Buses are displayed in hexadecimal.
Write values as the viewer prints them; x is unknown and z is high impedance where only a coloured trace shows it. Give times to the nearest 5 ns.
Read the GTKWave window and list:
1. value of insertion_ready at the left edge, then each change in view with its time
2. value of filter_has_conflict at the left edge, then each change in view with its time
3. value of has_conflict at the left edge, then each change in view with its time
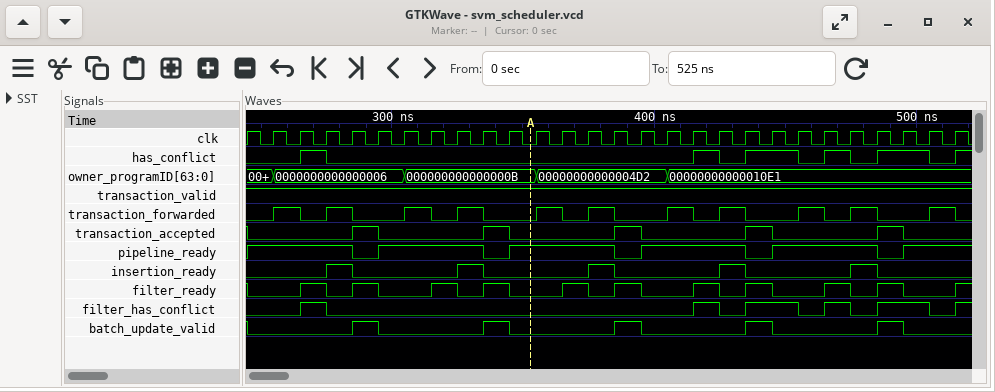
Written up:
0, 1 at 275 ns, 0 at 285 ns, 1 at 325 ns, 0 at 335 ns, 1 at 375 ns, 0 at 385 ns, 1 at 425 ns, 0 at 435 ns, 1 at 475 ns, 0 at 485 ns
0, 1 at 265 ns, 0 at 275 ns, 1 at 415 ns, 0 at 425 ns, 1 at 435 ns, 0 at 455 ns, 1 at 465 ns, 0 at 475 ns, 1 at 485 ns, 0 at 505 ns, 1 at 515 ns
0, 1 at 265 ns, 0 at 275 ns, 1 at 415 ns, 0 at 425 ns, 1 at 435 ns, 0 at 455 ns, 1 at 465 ns, 0 at 475 ns, 1 at 485 ns, 0 at 505 ns, 1 at 515 ns
